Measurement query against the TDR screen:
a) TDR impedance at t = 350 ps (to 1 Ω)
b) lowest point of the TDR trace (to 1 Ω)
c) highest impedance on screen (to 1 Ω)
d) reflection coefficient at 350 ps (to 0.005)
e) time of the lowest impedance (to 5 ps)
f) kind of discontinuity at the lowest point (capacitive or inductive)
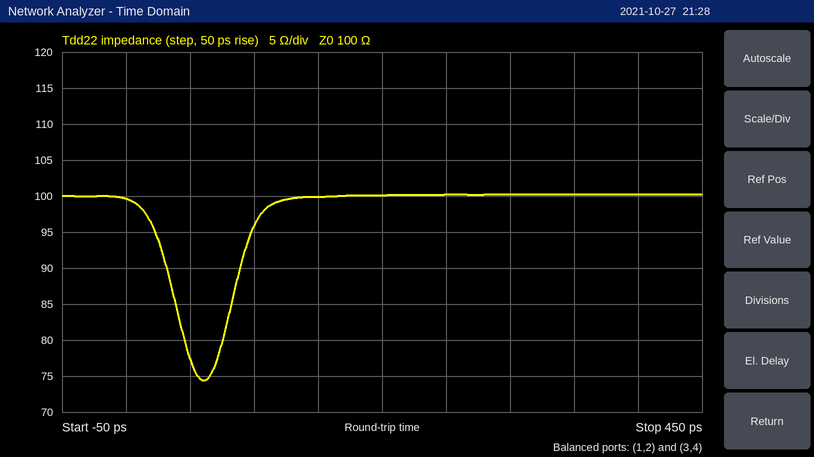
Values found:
100 Ω
74 Ω
100 Ω
0.000
60 ps
capacitive
